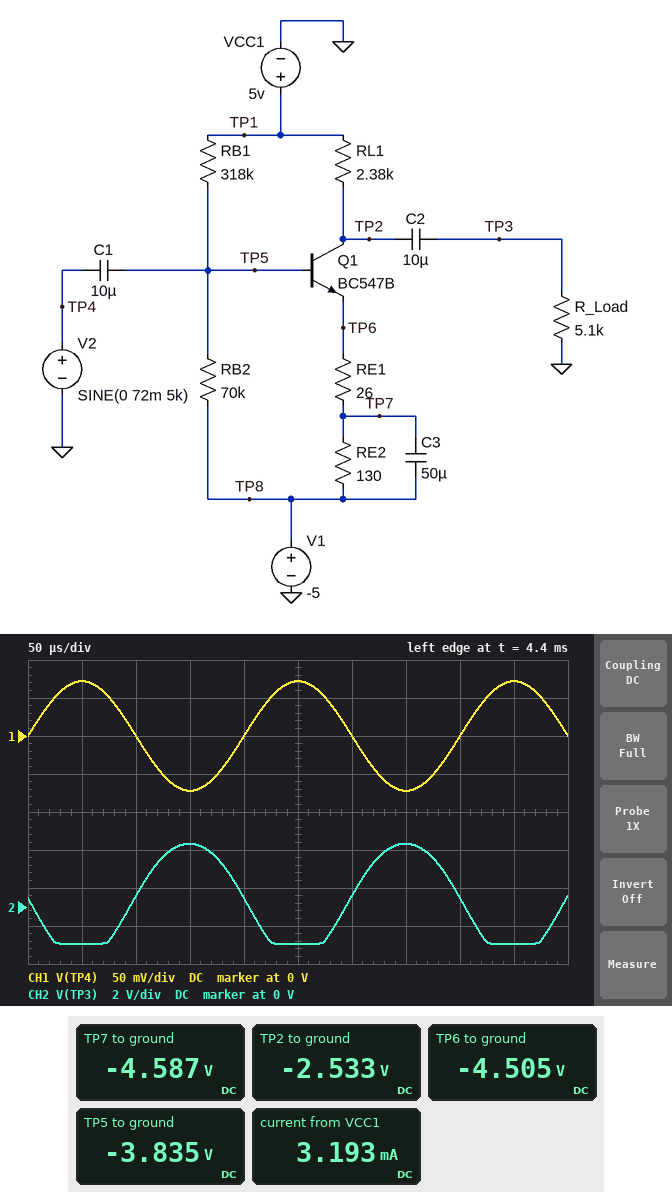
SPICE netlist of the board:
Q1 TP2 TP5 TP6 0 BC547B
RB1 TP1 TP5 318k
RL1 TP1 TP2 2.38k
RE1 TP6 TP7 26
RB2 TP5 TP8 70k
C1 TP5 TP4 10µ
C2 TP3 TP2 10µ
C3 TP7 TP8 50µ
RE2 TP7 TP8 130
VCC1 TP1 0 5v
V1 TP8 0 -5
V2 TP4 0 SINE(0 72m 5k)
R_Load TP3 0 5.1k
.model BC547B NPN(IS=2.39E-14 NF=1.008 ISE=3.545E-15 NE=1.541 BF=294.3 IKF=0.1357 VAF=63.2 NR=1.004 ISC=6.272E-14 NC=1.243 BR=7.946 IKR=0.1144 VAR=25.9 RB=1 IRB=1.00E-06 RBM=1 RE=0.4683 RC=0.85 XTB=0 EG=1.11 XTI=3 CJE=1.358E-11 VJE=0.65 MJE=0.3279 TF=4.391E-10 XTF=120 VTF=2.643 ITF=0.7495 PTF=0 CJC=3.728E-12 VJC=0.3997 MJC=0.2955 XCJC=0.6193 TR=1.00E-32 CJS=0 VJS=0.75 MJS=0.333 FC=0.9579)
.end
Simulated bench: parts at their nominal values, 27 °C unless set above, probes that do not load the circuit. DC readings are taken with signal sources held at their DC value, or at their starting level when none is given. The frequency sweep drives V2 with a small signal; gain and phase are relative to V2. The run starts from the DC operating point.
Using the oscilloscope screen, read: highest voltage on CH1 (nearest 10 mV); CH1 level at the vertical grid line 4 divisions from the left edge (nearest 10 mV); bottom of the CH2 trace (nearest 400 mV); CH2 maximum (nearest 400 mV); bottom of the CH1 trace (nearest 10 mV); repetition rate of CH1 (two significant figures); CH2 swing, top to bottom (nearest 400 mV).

70 mV
0 V
-2.0 V
3.2 V
-70 mV
5.0 kHz
5.2 V
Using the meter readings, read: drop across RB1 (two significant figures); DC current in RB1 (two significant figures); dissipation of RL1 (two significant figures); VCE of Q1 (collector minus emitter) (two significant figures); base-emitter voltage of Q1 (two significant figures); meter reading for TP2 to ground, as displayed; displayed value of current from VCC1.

8.8 V
28 µA
24 mW
2.0 V
670 mV
-2.533 V
3.193 mA
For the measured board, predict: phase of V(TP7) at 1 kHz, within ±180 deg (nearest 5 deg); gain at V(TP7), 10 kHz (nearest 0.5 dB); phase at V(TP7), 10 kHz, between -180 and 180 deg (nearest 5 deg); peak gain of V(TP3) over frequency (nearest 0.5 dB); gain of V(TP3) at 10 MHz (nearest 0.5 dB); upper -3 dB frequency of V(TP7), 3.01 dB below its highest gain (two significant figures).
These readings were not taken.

-85 deg
-41.0 dB
-90 deg
33.0 dB
33.0 dB
120 Hz
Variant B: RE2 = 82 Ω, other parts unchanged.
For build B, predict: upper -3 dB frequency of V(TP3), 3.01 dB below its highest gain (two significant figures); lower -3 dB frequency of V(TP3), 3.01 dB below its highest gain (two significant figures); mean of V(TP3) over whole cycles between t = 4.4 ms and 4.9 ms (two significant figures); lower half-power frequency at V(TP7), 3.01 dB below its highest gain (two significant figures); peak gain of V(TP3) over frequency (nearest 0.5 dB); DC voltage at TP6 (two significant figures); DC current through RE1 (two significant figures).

31 MHz
120 Hz
1.1 V
820 mHz
33.5 dB
-4.6 V
3.6 mA
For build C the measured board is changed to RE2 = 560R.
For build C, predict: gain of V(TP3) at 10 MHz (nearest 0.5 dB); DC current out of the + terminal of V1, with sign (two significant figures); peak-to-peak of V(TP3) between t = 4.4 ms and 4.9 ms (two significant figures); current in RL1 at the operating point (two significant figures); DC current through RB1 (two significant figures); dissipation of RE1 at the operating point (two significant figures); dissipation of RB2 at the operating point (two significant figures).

31.0 dB
-1.5 mA
4.7 V
1.5 mA
27 µA
58 µW
33 µW
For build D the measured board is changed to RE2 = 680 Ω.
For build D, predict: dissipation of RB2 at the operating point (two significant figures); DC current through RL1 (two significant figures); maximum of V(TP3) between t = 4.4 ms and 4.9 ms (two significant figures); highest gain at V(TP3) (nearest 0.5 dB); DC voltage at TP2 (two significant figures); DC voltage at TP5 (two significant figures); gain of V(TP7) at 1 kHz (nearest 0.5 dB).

35 µW
1.3 mA
1.8 V
30.5 dB
1.9 V
-3.4 V
-23.5 dB
